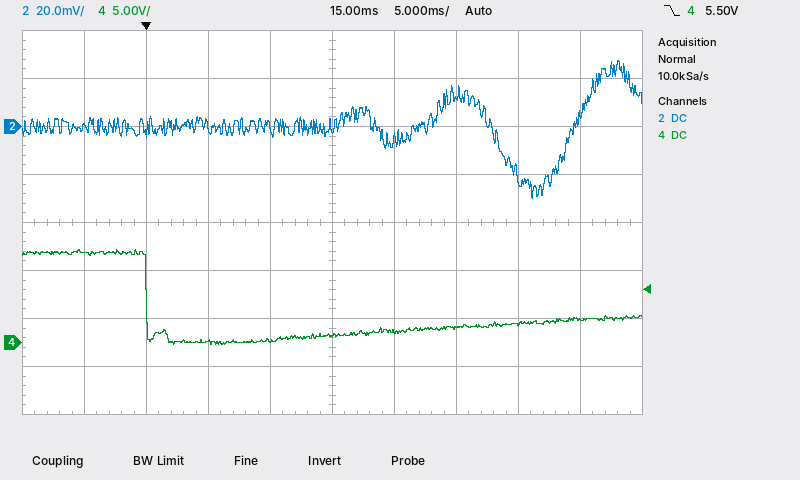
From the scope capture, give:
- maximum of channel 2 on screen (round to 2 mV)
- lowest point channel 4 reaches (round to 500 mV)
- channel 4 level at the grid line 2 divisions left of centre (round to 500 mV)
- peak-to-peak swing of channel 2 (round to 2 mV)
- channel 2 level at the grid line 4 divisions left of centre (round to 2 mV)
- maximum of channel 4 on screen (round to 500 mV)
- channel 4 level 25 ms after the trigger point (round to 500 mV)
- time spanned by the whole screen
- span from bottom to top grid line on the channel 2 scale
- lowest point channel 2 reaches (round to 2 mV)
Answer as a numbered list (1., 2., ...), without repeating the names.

1. 28 mV
2. 0.0 V
3. 0.0 V
4. 58 mV
5. 0 mV
6. 9.5 V
7. 1.5 V
8. 50 ms
9. 160 mV
10. -30 mV
